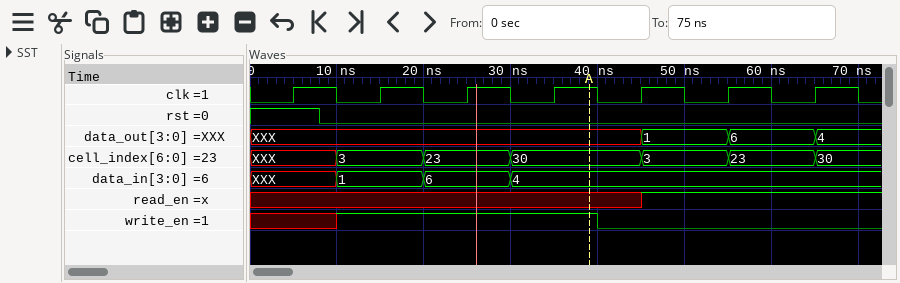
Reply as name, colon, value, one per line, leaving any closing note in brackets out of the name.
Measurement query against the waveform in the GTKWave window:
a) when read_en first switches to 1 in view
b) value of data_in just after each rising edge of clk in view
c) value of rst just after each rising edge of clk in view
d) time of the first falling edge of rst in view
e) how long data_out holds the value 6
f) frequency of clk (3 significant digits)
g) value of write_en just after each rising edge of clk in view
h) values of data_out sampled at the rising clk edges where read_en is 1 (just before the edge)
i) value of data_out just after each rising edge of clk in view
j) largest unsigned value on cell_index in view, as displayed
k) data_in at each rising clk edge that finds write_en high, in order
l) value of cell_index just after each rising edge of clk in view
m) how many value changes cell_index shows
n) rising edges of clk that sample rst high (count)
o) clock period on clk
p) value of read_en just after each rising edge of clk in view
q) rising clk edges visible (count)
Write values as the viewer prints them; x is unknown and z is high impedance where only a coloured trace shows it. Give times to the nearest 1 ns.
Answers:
when read_en first switches to 1 in view: 45 ns
value of data_in just after each rising edge of clk in view: XXX, 1, 6, 4, 4, 4, 4
value of rst just after each rising edge of clk in view: 1 0 0 0 0 0 0
time of the first falling edge of rst in view: 8 ns
how long data_out holds the value 6: 10 ns
frequency of clk: 100 MHz
value of write_en just after each rising edge of clk in view: x 1 1 1 0 0 0
values of data_out sampled at the rising clk edges where read_en is 1: 1, 6
value of data_out just after each rising edge of clk in view: XXX, XXX, XXX, XXX, 1, 6, 4
largest unsigned value on cell_index in view, as displayed: 30
data_in at each rising clk edge that finds write_en high, in order: 1, 6, 4
value of cell_index just after each rising edge of clk in view: XXX, 3, 23, 30, 3, 23, 30
how many value changes cell_index shows: 6
rising edges of clk that sample rst high: 1
clock period on clk: 10 ns
value of read_en just after each rising edge of clk in view: x x x x 1 1 1
rising clk edges visible: 7
